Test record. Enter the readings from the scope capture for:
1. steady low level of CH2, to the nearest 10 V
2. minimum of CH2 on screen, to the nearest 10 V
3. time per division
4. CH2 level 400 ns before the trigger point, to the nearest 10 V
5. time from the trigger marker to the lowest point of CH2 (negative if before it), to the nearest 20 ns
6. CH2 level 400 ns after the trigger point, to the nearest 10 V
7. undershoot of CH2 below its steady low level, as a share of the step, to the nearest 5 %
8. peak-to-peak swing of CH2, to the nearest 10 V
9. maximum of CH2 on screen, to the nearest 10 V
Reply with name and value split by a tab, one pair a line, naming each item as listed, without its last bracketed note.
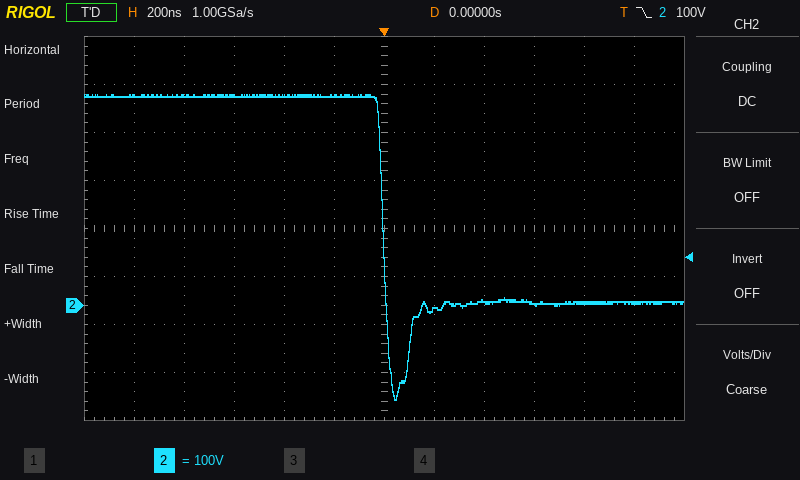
steady low level of CH2, to the nearest 10 V	10 V
minimum of CH2 on screen, to the nearest 10 V	-200 V
time per division	200 ns
CH2 level 400 ns before the trigger point, to the nearest 10 V	440 V
time from the trigger marker to the lowest point of CH2 (negative if before it), to the nearest 20 ns	+40 ns
CH2 level 400 ns after the trigger point, to the nearest 10 V	10 V
undershoot of CH2 below its steady low level, as a share of the step, to the nearest 5 %	45 %
peak-to-peak swing of CH2, to the nearest 10 V	640 V
maximum of CH2 on screen, to the nearest 10 V	440 V
